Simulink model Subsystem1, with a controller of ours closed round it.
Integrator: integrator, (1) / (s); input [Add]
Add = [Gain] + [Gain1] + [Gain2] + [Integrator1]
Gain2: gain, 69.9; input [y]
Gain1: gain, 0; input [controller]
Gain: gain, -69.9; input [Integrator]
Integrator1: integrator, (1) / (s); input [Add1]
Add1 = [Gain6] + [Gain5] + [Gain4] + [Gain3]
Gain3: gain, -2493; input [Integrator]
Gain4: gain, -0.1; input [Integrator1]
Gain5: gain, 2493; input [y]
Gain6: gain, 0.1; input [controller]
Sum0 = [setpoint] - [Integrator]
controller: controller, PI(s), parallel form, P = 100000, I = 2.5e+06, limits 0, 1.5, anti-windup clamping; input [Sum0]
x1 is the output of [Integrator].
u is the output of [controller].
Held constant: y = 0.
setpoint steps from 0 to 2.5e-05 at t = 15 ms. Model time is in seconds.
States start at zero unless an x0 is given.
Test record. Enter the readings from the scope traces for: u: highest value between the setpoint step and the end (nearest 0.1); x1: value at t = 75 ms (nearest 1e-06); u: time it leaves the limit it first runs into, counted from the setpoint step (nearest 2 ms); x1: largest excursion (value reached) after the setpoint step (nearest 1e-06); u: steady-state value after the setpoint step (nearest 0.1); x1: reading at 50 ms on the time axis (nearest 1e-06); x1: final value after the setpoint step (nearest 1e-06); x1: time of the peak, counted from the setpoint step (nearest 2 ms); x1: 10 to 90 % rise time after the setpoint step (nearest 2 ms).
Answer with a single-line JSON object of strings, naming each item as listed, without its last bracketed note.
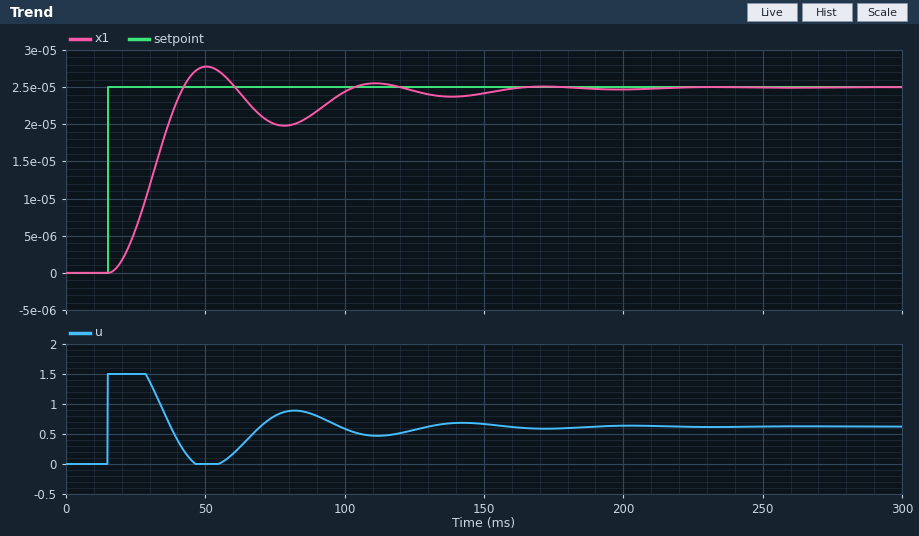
{"u: highest value between the setpoint step and the end": "1.5", "x1: value at t = 75 ms": "0.000020", "u: time it leaves the limit it first runs into, counted from the setpoint step": "14 ms", "x1: largest excursion (value reached) after the setpoint step": "0.000028", "u: steady-state value after the setpoint step": "0.6", "x1: reading at 50 ms on the time axis": "0.000028", "x1: final value after the setpoint step": "0.000025", "x1: time of the peak, counted from the setpoint step": "36 ms", "x1: 10 to 90 % rise time after the setpoint step": "18 ms"}
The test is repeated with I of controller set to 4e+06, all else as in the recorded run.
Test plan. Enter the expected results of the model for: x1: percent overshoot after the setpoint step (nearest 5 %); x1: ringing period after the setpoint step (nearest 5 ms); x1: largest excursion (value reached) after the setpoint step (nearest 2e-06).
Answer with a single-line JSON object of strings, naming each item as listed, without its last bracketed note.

{"x1: percent overshoot after the setpoint step": "15 %", "x1: ringing period after the setpoint step": "60 ms", "x1: largest excursion (value reached) after the setpoint step": "0.000028"}
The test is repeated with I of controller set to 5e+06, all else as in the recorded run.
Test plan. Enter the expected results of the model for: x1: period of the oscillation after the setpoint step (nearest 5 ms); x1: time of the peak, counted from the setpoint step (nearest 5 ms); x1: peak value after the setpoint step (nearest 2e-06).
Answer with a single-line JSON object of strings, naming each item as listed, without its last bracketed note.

{"x1: period of the oscillation after the setpoint step": "60 ms", "x1: time of the peak, counted from the setpoint step": "35 ms", "x1: peak value after the setpoint step": "0.000030"}
